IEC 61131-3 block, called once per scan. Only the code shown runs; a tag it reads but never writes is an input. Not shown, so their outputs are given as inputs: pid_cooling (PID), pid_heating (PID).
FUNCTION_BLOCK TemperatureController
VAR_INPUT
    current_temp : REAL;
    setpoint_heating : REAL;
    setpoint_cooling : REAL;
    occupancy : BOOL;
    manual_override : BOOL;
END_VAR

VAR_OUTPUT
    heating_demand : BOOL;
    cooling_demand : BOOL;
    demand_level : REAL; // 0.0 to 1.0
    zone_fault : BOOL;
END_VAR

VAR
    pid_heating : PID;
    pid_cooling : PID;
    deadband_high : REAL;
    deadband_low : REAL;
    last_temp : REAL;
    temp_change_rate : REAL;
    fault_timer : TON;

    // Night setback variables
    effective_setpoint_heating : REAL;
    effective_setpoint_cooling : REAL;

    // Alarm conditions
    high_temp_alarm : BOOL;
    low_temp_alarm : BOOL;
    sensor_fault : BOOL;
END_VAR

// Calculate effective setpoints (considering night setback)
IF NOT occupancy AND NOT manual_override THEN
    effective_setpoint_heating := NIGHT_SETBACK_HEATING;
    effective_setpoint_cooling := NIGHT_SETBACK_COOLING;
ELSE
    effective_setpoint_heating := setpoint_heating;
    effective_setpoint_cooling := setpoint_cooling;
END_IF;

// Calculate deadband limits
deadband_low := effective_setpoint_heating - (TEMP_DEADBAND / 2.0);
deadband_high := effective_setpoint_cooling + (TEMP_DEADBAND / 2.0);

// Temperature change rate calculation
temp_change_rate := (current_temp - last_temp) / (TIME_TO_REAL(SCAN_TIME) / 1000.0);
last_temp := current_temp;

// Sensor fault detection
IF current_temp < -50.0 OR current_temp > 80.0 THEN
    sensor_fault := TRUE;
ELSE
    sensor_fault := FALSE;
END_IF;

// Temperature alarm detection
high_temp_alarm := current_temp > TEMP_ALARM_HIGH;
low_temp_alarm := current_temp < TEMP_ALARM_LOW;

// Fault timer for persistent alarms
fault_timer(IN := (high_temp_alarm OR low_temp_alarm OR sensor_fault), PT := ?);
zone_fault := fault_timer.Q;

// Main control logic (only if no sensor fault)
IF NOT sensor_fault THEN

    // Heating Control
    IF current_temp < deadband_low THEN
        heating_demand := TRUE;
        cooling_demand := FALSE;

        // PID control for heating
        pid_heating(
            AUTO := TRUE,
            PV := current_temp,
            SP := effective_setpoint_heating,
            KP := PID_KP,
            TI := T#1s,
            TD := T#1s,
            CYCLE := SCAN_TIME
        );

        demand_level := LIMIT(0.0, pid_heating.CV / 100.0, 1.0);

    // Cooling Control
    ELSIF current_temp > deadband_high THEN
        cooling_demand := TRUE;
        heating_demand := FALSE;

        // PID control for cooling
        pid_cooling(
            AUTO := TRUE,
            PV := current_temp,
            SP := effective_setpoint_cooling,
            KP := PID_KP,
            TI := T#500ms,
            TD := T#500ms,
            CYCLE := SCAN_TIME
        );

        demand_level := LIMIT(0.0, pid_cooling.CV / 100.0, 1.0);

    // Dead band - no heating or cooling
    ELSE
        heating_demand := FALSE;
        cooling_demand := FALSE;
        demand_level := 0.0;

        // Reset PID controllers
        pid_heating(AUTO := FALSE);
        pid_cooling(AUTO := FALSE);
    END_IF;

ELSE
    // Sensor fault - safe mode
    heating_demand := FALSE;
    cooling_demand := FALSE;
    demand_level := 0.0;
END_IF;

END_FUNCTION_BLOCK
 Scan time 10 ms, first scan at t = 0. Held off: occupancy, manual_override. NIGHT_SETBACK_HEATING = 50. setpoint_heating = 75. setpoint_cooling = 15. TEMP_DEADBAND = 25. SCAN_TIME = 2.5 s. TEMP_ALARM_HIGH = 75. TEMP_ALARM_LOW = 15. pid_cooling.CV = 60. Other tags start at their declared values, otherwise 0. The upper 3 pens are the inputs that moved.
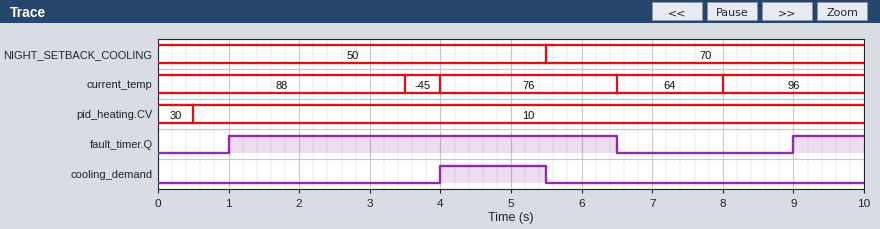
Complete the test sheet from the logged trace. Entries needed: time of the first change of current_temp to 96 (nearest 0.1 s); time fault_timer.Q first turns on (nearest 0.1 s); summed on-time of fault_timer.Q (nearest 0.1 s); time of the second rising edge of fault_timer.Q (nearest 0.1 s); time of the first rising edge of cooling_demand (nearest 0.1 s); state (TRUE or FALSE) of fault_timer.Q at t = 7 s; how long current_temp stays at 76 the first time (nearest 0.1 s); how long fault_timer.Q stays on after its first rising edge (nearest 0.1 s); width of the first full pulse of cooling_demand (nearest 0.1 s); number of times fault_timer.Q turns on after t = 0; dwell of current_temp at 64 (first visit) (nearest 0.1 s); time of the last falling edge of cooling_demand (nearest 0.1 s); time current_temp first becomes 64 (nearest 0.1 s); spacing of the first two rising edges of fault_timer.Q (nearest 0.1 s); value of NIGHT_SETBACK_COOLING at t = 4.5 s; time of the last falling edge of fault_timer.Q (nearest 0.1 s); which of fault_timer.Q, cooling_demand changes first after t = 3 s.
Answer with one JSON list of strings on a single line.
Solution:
["8.0 s", "1.0 s", "6.5 s", "9.0 s", "4.0 s", "FALSE", "2.5 s", "5.5 s", "1.5 s", "2", "1.5 s", "5.5 s", "6.5 s", "8.0 s", "50", "6.5 s", "cooling_demand"]
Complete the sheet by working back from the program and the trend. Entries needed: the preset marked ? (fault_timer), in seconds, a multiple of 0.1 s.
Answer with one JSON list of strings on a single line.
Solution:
["1.0 s"]
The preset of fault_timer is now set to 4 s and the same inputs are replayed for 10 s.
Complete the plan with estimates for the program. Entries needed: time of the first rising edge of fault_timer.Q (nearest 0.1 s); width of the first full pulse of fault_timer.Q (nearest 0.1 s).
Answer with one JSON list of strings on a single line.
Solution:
["4.0 s", "2.5 s"]
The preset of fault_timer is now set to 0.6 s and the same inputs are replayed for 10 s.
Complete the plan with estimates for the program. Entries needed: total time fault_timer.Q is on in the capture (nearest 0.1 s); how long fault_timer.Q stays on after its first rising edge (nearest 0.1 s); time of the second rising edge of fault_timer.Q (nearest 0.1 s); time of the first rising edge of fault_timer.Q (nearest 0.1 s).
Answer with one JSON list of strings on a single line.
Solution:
["7.3 s", "5.9 s", "8.6 s", "0.6 s"]
